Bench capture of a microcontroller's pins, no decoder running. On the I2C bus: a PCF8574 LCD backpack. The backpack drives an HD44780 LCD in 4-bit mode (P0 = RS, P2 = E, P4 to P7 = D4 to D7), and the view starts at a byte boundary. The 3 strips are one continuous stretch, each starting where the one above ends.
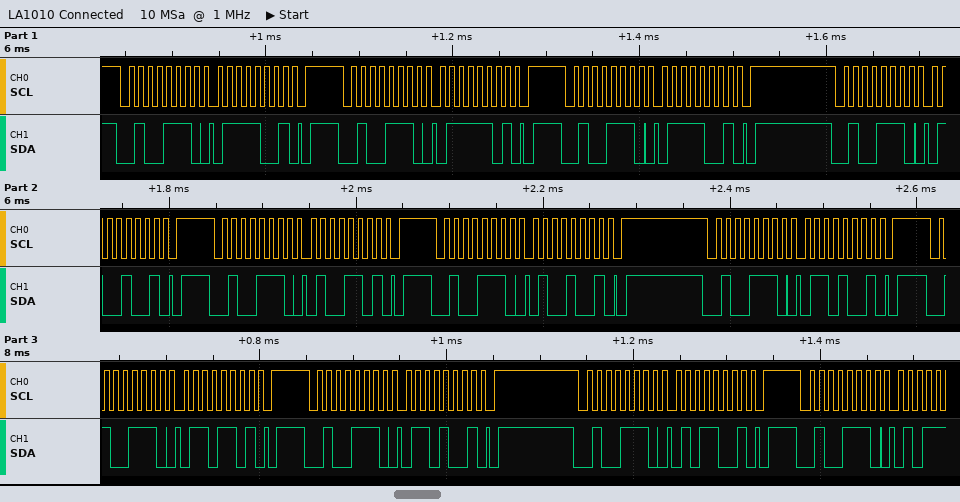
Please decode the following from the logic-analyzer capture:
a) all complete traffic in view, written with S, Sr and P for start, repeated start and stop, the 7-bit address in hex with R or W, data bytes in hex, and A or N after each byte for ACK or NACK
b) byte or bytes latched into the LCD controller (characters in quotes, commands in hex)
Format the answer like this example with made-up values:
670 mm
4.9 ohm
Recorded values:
S 27W A 79 A P S 27W A 7D A P S 27W A 79 A P S 27W A 49 A P S 27W A 4D A P S 27W A 49 A P S 27W A 69 A P S 27W A 6D A P S 27W A 69 A P S 27W A 59 A P S 27W A
't'
